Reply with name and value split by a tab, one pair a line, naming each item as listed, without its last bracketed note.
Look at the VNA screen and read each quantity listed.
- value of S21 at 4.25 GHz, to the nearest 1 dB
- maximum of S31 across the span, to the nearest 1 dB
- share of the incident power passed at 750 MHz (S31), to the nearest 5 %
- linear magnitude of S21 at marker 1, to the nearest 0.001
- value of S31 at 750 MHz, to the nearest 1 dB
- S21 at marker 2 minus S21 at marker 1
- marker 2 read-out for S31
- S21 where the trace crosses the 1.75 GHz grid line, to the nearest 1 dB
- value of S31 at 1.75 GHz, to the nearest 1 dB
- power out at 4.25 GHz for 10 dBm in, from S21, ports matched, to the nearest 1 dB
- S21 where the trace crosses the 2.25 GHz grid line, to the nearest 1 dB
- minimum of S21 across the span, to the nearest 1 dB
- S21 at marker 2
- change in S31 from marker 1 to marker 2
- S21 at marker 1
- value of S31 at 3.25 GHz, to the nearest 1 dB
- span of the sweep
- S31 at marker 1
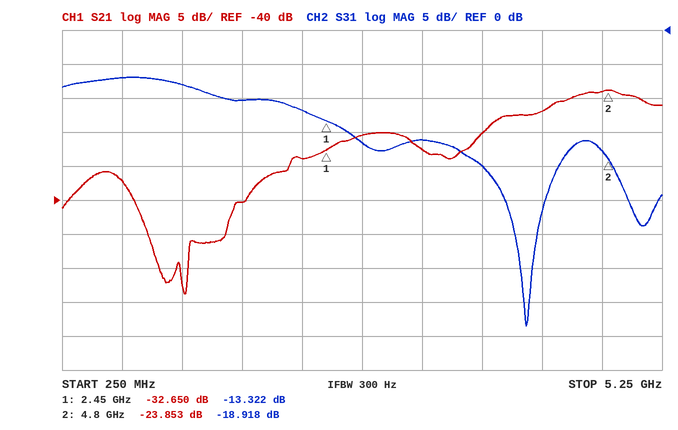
value of S21 at 4.25 GHz, to the nearest 1 dB	-27 dB
maximum of S31 across the span, to the nearest 1 dB	-7 dB
share of the incident power passed at 750 MHz (S31), to the nearest 5 %	20 %
linear magnitude of S21 at marker 1, to the nearest 0.001	0.023
value of S31 at 750 MHz, to the nearest 1 dB	-7 dB
S21 at marker 2 minus S21 at marker 1	8.797 dB
marker 2 read-out for S31	-18.918 dB
S21 where the trace crosses the 1.75 GHz grid line, to the nearest 1 dB	-40 dB
value of S31 at 1.75 GHz, to the nearest 1 dB	-10 dB
power out at 4.25 GHz for 10 dBm in, from S21, ports matched, to the nearest 1 dB	-17 dBm
S21 where the trace crosses the 2.25 GHz grid line, to the nearest 1 dB	-34 dB
minimum of S21 across the span, to the nearest 1 dB	-54 dB
S21 at marker 2	-23.853 dB
change in S31 from marker 1 to marker 2	-5.596 dB
S21 at marker 1	-32.650 dB
value of S31 at 3.25 GHz, to the nearest 1 dB	-16 dB
span of the sweep	5 GHz
S31 at marker 1	-13.322 dB
